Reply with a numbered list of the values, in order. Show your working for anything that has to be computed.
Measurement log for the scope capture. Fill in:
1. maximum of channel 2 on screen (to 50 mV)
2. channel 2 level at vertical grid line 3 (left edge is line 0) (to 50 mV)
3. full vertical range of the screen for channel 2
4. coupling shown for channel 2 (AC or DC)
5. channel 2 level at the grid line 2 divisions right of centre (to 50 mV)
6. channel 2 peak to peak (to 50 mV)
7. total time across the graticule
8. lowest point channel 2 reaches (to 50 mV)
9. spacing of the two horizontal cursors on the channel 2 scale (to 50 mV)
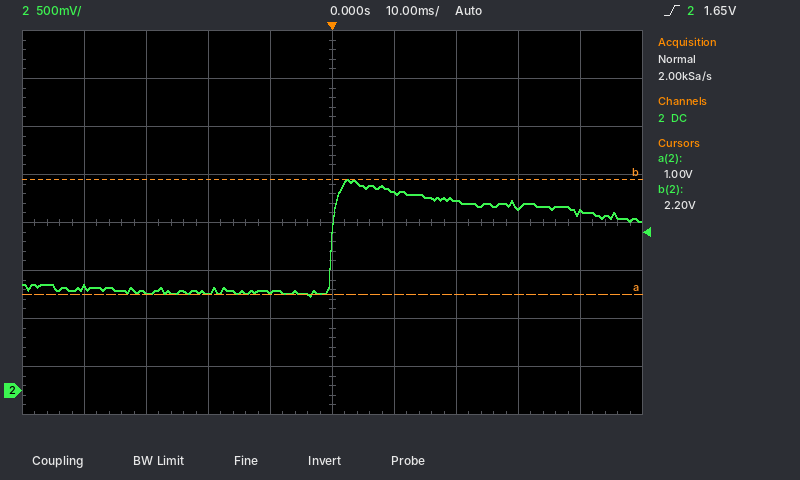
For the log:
1. 2.20 V
2. 1.00 V
3. 4 V
4. DC
5. 2.00 V
6. 2.20 V − (1.00 V) = 1.20 V
7. 100 ms
8. 1.00 V
9. 1.20 V
